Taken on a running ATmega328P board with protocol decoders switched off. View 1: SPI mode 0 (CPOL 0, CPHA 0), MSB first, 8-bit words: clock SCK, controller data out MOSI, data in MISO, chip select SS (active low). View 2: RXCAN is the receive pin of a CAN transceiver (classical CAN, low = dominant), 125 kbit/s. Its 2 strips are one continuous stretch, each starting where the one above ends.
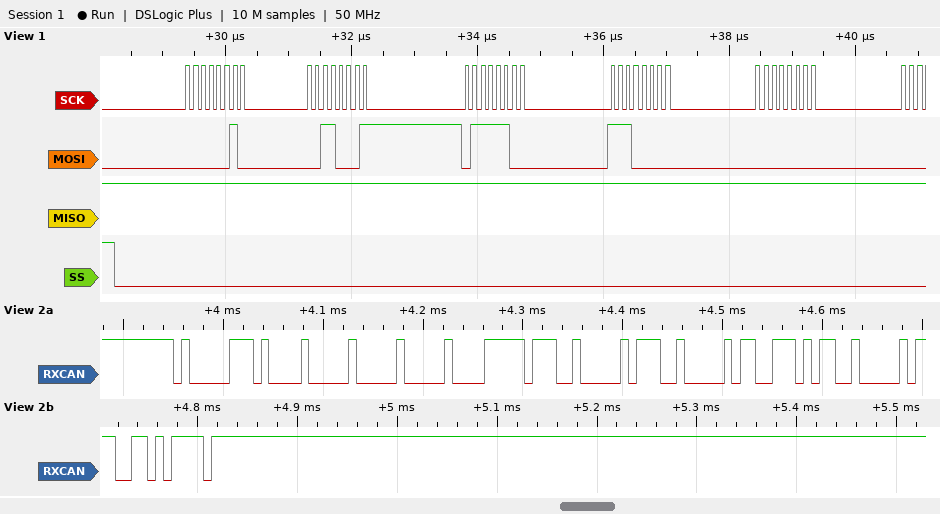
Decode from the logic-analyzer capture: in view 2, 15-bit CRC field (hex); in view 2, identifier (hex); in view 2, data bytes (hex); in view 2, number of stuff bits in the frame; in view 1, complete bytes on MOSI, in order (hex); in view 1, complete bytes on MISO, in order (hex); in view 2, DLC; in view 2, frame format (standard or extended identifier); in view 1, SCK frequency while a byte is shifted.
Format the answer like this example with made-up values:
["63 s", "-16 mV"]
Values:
["0x1CD7", "0x41A", "00 00 FF 20 72 06 75 90", "8", "02 31 7C E0 00", "FF FF FF FF FF", "8", "standard", "8 MHz"]
